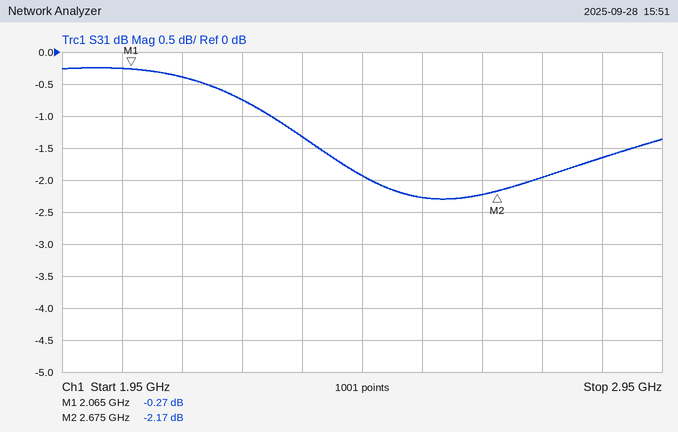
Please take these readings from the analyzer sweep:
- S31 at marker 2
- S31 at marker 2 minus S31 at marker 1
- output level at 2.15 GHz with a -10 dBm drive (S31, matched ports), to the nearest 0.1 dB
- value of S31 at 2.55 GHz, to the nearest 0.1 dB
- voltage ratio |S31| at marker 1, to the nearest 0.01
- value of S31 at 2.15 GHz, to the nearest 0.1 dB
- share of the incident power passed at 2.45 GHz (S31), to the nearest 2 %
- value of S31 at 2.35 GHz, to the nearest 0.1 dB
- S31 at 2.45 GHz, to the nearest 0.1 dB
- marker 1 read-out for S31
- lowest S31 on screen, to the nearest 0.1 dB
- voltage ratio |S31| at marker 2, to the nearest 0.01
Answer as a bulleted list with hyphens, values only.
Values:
- -2.17 dB
- -1.90 dB
- -10.4 dBm
- -2.3 dB
- 0.97
- -0.4 dB
- 64 %
- -1.3 dB
- -1.9 dB
- -0.27 dB
- -2.3 dB
- 0.78
